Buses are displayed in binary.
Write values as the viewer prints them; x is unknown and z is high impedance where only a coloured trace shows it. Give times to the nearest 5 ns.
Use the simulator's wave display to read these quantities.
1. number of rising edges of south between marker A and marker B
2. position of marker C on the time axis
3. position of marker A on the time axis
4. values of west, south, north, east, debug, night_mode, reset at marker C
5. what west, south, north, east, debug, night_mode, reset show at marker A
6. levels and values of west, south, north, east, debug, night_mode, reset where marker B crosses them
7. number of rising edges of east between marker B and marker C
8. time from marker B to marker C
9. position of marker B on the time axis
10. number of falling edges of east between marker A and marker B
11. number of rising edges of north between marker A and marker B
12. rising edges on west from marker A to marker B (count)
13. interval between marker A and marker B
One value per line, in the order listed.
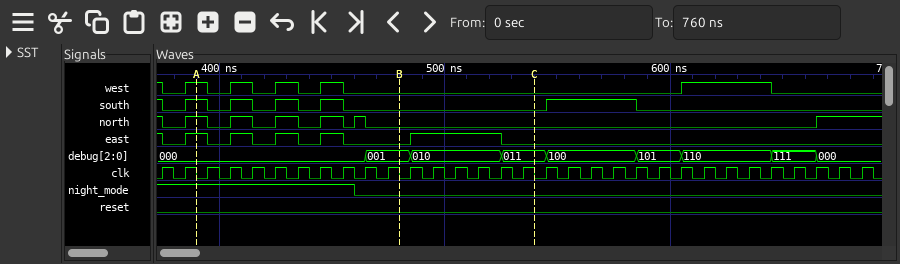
3
540 ns
390 ns
west=0, south=0, north=0, east=0, debug=011, night_mode=0, reset=0
west=1, south=1, north=1, east=1, debug=000, night_mode=1, reset=0
west=0, south=0, north=0, east=0, debug=001, night_mode=0, reset=0
1
60 ns
480 ns
4
4
3
90 ns
